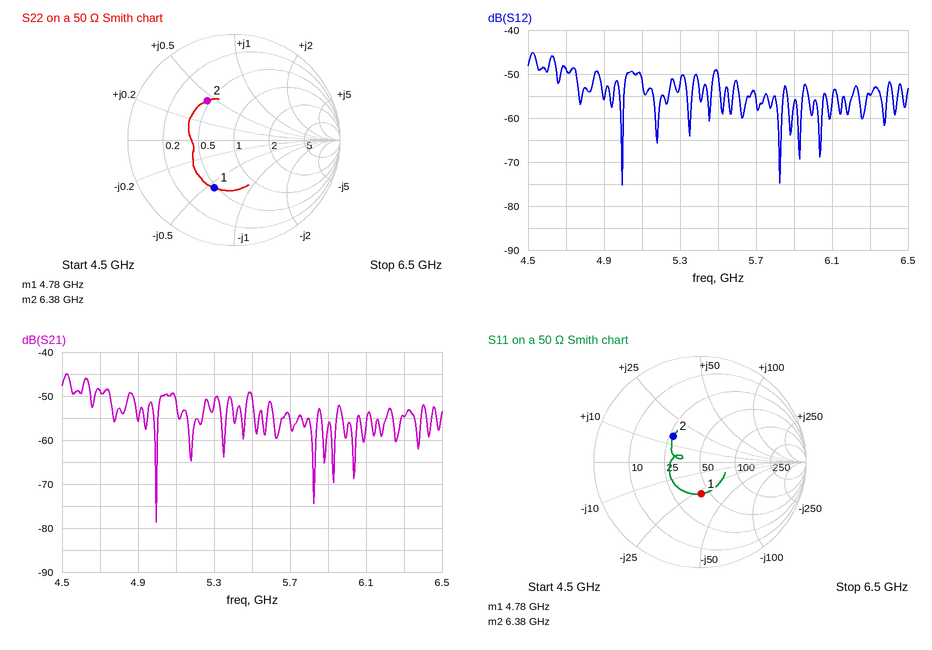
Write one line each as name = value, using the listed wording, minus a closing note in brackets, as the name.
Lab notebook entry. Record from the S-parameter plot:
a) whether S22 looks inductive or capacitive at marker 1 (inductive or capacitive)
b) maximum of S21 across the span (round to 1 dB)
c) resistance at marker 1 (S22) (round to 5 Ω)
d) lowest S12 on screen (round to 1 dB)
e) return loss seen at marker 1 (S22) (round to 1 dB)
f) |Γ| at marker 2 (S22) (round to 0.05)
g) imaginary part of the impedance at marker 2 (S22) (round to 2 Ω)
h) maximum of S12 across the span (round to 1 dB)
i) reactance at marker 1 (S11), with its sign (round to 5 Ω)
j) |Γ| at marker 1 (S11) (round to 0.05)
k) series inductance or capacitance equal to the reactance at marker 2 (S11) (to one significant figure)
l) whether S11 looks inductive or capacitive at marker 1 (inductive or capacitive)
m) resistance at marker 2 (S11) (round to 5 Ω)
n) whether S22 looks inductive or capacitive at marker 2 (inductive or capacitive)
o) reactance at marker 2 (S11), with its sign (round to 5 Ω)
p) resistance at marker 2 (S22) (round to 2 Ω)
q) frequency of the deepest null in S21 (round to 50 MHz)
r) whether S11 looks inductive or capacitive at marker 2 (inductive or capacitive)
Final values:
whether S22 looks inductive or capacitive at marker 1 = capacitive
maximum of S21 across the span = -45 dB
resistance at marker 1 (S22) = 25 Ω
lowest S12 on screen = -75 dB
return loss seen at marker 1 (S22) = 6 dB
|Γ| at marker 2 (S22) = 0.45
imaginary part of the impedance at marker 2 (S22) = +22 Ω
maximum of S12 across the span = -45 dB
reactance at marker 1 (S11), with its sign = -30 Ω
|Γ| at marker 1 (S11) = 0.30
series inductance or capacitance equal to the reactance at marker 2 (S11) = 400 pH
whether S11 looks inductive or capacitive at marker 1 = capacitive
resistance at marker 2 (S11) = 25 Ω
whether S22 looks inductive or capacitive at marker 2 = inductive
reactance at marker 2 (S11), with its sign = +15 Ω
resistance at marker 2 (S22) = 24 Ω
frequency of the deepest null in S21 = 5.00 GHz
whether S11 looks inductive or capacitive at marker 2 = inductive
